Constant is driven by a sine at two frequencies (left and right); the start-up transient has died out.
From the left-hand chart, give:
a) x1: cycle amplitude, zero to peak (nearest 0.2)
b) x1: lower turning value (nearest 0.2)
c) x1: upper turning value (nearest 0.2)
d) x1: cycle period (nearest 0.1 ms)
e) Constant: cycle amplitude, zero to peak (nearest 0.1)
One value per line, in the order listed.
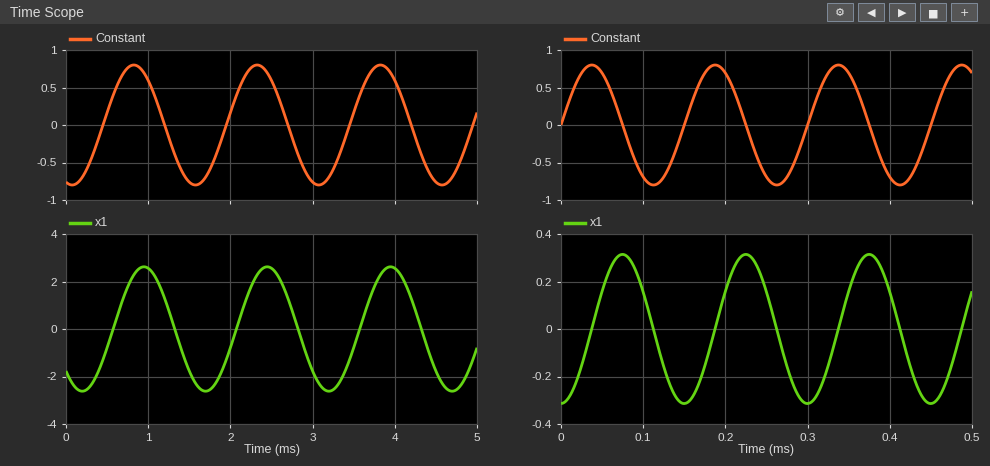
2.6
-2.6
2.6
1.5 ms
0.8
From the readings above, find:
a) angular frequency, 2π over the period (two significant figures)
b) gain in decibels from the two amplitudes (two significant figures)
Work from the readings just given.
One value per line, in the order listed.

4.2 rad/ms
10 dB
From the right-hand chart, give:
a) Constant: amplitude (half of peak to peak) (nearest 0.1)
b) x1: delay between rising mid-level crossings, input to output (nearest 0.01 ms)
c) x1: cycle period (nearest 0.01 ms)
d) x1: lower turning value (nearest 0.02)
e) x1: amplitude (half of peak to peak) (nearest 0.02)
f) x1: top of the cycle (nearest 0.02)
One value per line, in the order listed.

0.8
0.04 ms
0.15 ms
-0.32
0.32
0.32
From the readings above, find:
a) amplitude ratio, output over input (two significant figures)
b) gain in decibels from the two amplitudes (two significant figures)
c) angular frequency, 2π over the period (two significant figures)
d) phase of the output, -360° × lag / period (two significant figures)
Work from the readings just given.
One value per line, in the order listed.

0.40
-8.0 dB
42 rad/ms
-96°
